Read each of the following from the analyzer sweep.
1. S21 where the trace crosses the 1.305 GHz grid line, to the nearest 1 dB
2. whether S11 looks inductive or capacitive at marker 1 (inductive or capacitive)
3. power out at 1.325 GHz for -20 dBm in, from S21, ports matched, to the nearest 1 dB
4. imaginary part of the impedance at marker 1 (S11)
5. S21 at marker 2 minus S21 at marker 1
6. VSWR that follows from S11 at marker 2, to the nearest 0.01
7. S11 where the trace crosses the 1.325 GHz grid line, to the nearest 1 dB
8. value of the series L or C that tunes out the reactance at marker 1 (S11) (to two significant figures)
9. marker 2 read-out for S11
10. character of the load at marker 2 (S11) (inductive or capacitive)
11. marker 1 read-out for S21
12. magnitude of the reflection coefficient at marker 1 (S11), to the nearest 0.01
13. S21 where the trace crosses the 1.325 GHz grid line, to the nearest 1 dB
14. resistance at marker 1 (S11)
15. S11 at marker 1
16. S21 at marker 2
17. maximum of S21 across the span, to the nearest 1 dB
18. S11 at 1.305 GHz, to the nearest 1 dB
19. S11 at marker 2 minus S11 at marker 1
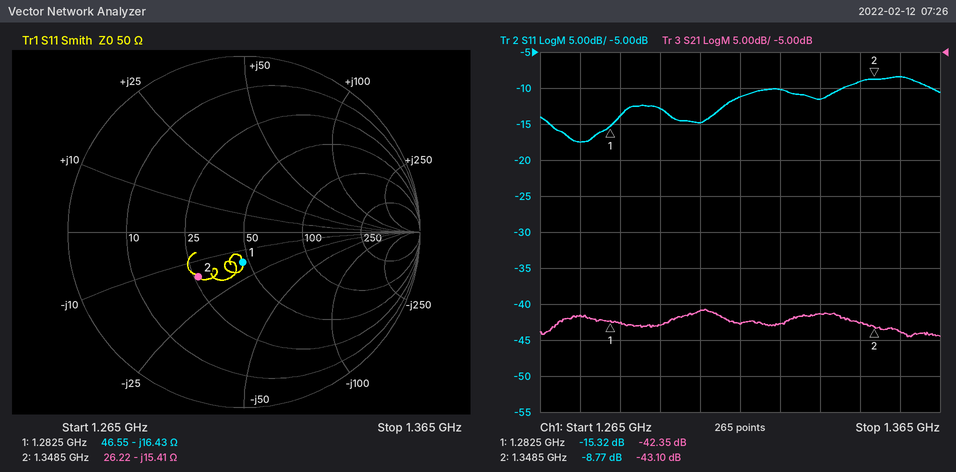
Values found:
-41 dB
capacitive
-63 dBm
-16.43 Ω
-0.75 dB
2.15
-10 dB
2.0 nH
-8.77 dB
capacitive
-42.35 dB
0.17
-43 dB
46.55 Ω
-15.32 dB
-43.10 dB
-41 dB
-15 dB
6.55 dB
